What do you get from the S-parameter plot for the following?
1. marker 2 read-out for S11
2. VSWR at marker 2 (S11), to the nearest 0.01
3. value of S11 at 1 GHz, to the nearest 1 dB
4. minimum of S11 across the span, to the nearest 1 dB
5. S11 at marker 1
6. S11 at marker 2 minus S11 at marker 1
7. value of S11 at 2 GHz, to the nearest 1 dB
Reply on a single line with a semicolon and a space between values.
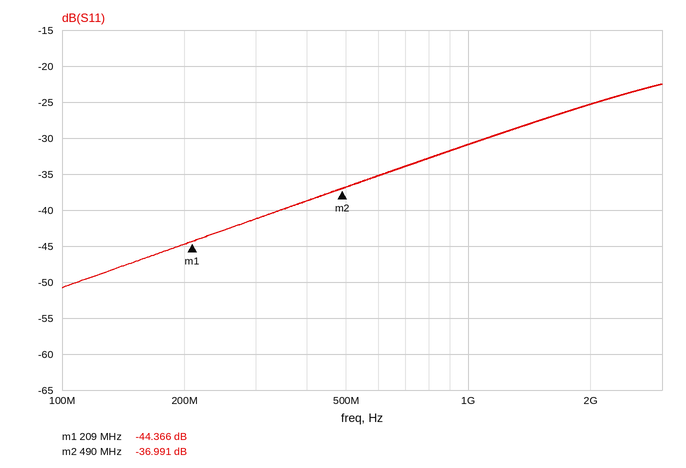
-36.991 dB; 1.03; -31 dB; -51 dB; -44.366 dB; 7.375 dB; -25 dB
